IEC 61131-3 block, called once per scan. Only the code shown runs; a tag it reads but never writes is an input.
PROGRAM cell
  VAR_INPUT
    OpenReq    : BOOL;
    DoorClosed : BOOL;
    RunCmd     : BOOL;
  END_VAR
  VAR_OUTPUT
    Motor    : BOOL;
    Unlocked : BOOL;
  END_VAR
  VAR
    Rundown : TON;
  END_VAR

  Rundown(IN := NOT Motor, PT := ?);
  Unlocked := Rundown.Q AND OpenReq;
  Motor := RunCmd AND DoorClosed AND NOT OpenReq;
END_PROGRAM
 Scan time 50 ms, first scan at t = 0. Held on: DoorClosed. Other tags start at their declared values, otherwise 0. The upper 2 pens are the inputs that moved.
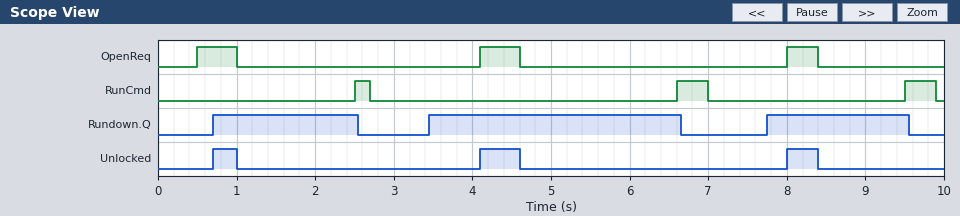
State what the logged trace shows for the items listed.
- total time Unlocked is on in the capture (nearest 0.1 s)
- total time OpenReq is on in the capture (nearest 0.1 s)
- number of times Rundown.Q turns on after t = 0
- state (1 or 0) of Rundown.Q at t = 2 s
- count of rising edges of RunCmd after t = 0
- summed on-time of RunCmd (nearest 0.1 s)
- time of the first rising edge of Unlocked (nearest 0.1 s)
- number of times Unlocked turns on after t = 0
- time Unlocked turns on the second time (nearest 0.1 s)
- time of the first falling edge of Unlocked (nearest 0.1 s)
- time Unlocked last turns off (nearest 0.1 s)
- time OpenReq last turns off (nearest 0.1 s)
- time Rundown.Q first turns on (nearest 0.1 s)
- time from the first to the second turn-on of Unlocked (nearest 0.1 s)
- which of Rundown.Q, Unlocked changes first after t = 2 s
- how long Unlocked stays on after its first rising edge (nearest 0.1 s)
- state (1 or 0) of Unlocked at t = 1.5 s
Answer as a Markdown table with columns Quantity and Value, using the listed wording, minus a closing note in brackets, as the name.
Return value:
| Quantity | Value |
|---|---|
| total time Unlocked is on in the capture | 1.2 s |
| total time OpenReq is on in the capture | 1.4 s |
| number of times Rundown.Q turns on after t = 0 | 3 |
| state (1 or 0) of Rundown.Q at t = 2 s | 1 |
| count of rising edges of RunCmd after t = 0 | 3 |
| summed on-time of RunCmd | 1.0 s |
| time of the first rising edge of Unlocked | 0.7 s |
| number of times Unlocked turns on after t = 0 | 3 |
| time Unlocked turns on the second time | 4.1 s |
| time of the first falling edge of Unlocked | 1.0 s |
| time Unlocked last turns off | 8.4 s |
| time OpenReq last turns off | 8.4 s |
| time Rundown.Q first turns on | 0.7 s |
| time from the first to the second turn-on of Unlocked | 3.4 s |
| which of Rundown.Q, Unlocked changes first after t = 2 s | Rundown.Q |
| how long Unlocked stays on after its first rising edge | 0.3 s |
| state (1 or 0) of Unlocked at t = 1.5 s | 0 |
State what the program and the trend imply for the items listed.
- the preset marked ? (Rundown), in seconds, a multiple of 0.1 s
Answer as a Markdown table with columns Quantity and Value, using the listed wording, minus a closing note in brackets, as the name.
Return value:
| Quantity | Value |
|---|---|
| the preset marked ? (Rundown), in seconds, a multiple of 0.1 s | 0.7 s |
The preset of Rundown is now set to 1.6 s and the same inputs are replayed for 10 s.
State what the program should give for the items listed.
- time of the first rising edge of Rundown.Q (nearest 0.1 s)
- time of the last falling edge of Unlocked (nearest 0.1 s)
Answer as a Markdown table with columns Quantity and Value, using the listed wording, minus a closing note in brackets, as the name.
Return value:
| Quantity | Value |
|---|---|
| time of the first rising edge of Rundown.Q | 1.6 s |
| time of the last falling edge of Unlocked | 4.6 s |
